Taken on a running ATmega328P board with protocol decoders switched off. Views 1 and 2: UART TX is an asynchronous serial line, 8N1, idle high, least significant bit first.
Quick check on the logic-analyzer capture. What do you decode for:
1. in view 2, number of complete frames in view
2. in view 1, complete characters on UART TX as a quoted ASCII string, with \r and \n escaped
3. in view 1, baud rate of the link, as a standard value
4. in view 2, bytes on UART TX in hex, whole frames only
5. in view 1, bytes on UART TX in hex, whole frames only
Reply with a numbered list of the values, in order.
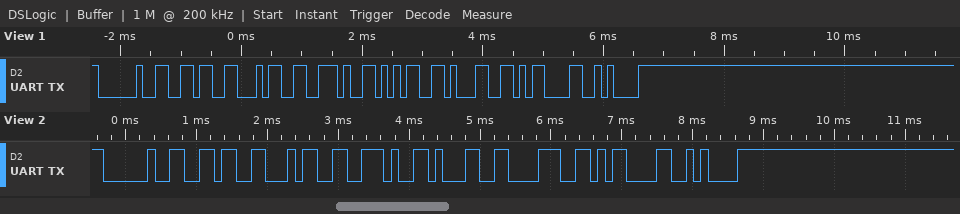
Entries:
1. 8
2. " 64.51\r\n"
3. 9600 baud
4. 0x20 0x36 0x34 0x2E 0x31 0x38 0x0D 0x0A
5. 20 36 34 2E 35 31 0D 0A
